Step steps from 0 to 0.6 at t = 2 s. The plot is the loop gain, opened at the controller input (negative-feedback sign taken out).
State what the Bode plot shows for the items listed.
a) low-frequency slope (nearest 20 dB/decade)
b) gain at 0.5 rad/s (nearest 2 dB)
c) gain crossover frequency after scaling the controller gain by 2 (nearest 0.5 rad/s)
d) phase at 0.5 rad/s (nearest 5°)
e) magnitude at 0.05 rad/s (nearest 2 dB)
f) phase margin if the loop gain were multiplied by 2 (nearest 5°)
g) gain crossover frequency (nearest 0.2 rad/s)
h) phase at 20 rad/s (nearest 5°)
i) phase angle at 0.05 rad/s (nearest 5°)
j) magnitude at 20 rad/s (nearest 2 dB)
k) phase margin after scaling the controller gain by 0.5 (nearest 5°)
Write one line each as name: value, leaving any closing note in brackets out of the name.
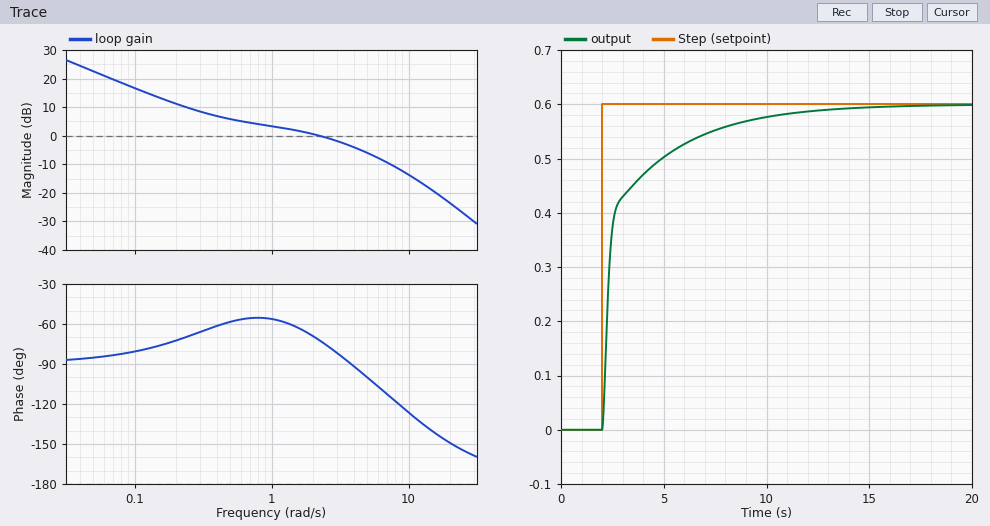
low-frequency slope: -20 dB/decade
gain at 0.5 rad/s: 6 dB
gain crossover frequency after scaling the controller gain by 2: 5.0 rad/s
phase at 0.5 rad/s: -60°
magnitude at 0.05 rad/s: 22 dB
phase margin if the loop gain were multiplied by 2: 80°
gain crossover frequency: 2.2 rad/s
phase at 20 rad/s: -150°
phase angle at 0.05 rad/s: -85°
magnitude at 20 rad/s: -24 dB
phase margin after scaling the controller gain by 0.5: 120°
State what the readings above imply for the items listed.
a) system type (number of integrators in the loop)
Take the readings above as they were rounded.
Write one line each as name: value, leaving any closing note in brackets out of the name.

system type: 1
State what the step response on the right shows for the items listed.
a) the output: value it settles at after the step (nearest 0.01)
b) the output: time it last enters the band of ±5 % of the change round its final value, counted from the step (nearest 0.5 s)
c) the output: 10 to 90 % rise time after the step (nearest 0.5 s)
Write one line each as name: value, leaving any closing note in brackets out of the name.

the output: value it settles at after the step: 0.60
the output: time it last enters the band of ±5 % of the change round its final value, counted from the step: 7.0 s
the output: 10 to 90 % rise time after the step: 4.5 s
